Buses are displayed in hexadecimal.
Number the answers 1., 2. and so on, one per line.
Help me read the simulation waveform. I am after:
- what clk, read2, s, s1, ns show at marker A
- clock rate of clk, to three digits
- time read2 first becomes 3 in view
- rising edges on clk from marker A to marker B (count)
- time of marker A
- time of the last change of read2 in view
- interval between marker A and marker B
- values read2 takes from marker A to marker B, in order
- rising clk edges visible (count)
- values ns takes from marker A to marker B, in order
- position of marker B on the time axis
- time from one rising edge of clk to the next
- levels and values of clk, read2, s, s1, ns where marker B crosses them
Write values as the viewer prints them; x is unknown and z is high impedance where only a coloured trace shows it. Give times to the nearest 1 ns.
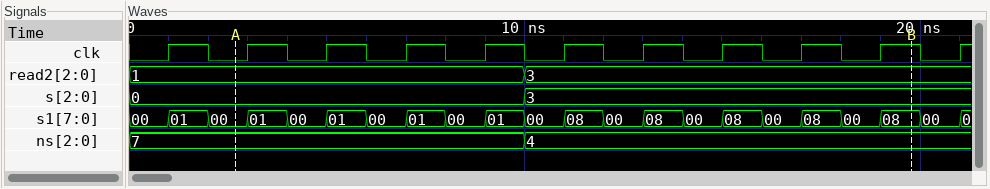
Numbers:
1. clk=0, read2=1, s=0, s1=00, ns=7
2. 500 MHz
3. 10 ns
4. 9
5. 3 ns
6. 10 ns
7. 17 ns
8. 1, 3
9. 11
10. 7, 4
11. 20 ns
12. 2 ns
13. clk=1, read2=3, s=3, s1=08, ns=4
